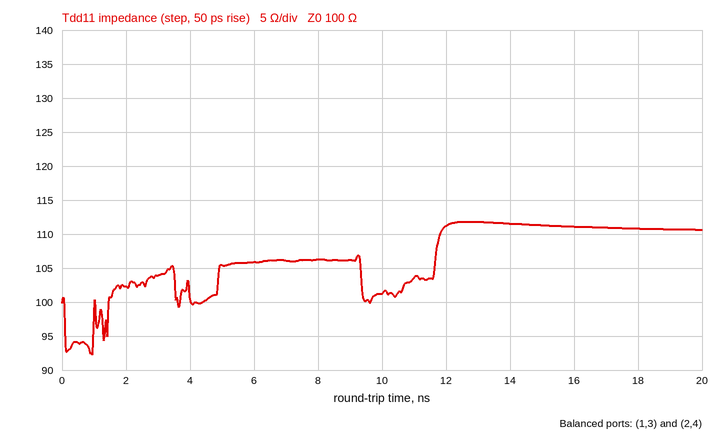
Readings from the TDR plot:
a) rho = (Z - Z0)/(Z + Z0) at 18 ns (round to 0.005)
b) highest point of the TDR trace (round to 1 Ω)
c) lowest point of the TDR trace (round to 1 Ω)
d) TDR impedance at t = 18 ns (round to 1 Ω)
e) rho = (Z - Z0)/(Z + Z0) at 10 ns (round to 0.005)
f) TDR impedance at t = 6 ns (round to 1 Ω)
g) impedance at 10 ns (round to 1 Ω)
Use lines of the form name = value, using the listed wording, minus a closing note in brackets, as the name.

rho = (Z - Z0)/(Z + Z0) at 18 ns = +0.050
highest point of the TDR trace = 112 Ω
lowest point of the TDR trace = 92 Ω
TDR impedance at t = 18 ns = 111 Ω
rho = (Z - Z0)/(Z + Z0) at 10 ns = +0.005
TDR impedance at t = 6 ns = 106 Ω
impedance at 10 ns = 101 Ω
